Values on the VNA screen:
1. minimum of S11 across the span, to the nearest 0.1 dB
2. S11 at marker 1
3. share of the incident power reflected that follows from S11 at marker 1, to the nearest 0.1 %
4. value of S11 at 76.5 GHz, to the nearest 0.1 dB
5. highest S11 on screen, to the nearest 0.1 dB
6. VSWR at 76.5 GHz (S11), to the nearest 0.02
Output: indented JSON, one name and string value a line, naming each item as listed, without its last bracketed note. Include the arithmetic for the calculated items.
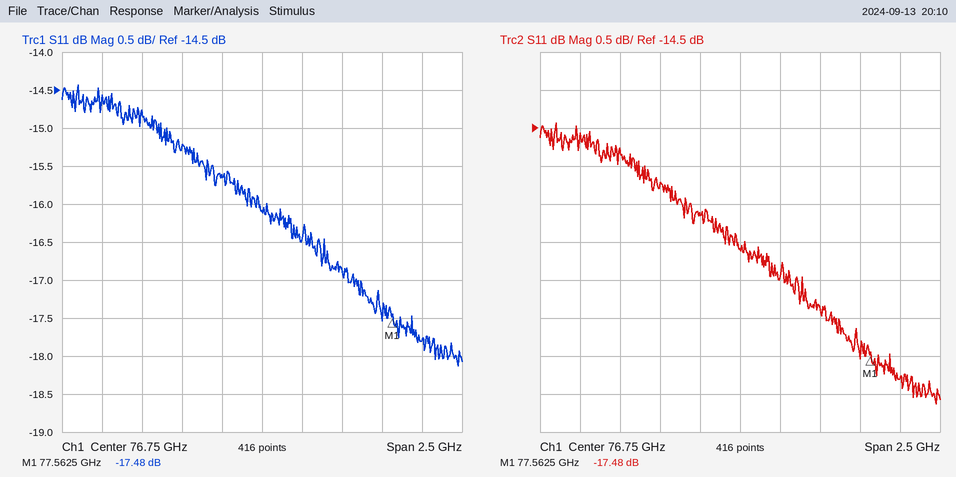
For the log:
{
  "minimum of S11 across the span, to the nearest 0.1 dB": "-18.1 dB",
  "S11 at marker 1": "-17.48 dB",
  "share of the incident power reflected that follows from S11 at marker 1, to the nearest 0.1 %": "10^(-17.48/10) ≈ 1.8 %",
  "value of S11 at 76.5 GHz, to the nearest 0.1 dB": "-15.6 dB",
  "highest S11 on screen, to the nearest 0.1 dB": "-14.4 dB",
  "VSWR at 76.5 GHz (S11), to the nearest 0.02": "|Γ| = 10^(-15.6/20) = 0.1660; VSWR = (1 + 0.1660)/(1 − 0.1660) ≈ 1.40"
}
